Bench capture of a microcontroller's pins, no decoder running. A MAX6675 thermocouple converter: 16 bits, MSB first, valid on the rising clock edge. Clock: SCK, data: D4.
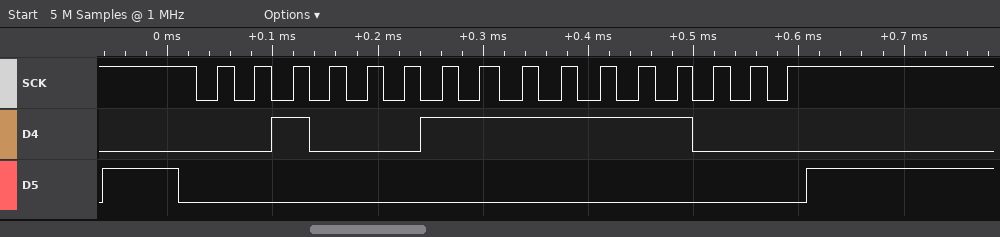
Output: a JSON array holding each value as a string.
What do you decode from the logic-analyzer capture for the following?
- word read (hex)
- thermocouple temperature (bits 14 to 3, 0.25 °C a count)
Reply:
["0x23F8", "287.75 °C"]
